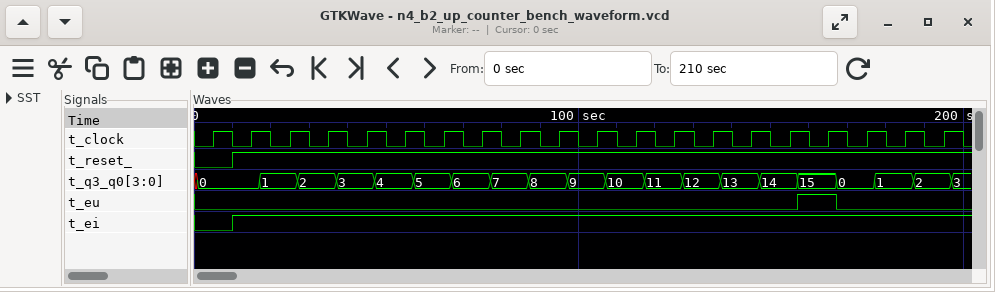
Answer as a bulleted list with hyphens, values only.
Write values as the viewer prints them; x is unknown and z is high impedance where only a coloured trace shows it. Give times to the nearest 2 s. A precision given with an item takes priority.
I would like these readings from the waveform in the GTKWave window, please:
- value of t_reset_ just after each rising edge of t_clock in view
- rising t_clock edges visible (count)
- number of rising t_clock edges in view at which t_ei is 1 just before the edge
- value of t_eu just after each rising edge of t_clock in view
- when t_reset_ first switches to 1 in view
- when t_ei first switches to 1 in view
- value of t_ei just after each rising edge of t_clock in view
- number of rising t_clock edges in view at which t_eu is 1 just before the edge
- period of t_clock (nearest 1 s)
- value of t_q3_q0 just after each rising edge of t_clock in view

- 0 1 1 1 1 1 1 1 1 1 1 1 1 1 1 1 1 1 1 1
- 20
- 19
- 0 0 0 0 0 0 0 0 0 0 0 0 0 0 0 0 1 0 0 0
- 10 s
- 10 s
- 0 1 1 1 1 1 1 1 1 1 1 1 1 1 1 1 1 1 1 1
- 1
- 10 s
- 0, 0, 1, 2, 3, 4, 5, 6, 7, 8, 9, 10, 11, 12, 13, 14, 15, 0, 1, 2
